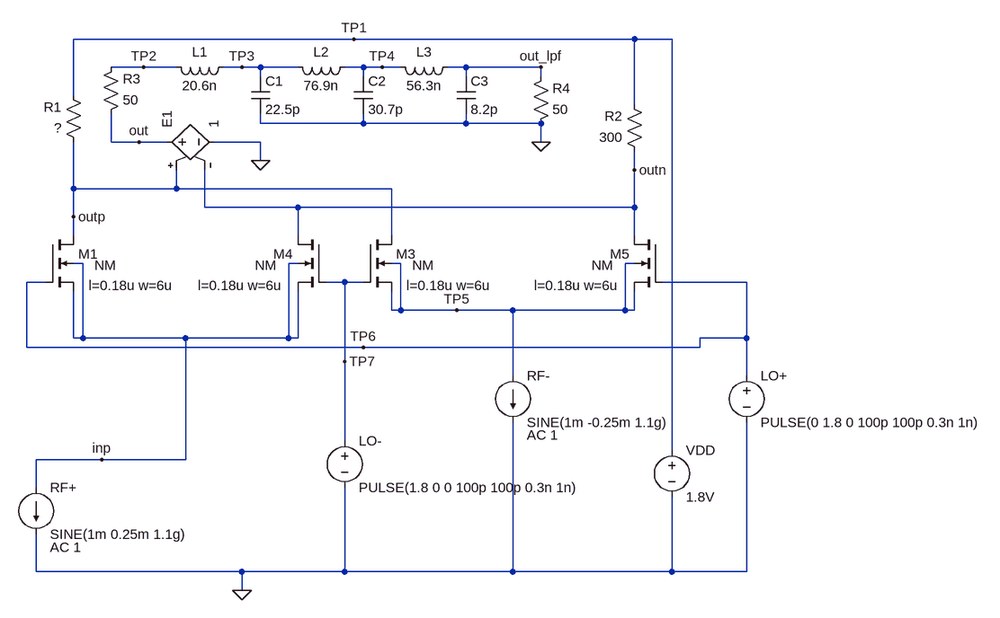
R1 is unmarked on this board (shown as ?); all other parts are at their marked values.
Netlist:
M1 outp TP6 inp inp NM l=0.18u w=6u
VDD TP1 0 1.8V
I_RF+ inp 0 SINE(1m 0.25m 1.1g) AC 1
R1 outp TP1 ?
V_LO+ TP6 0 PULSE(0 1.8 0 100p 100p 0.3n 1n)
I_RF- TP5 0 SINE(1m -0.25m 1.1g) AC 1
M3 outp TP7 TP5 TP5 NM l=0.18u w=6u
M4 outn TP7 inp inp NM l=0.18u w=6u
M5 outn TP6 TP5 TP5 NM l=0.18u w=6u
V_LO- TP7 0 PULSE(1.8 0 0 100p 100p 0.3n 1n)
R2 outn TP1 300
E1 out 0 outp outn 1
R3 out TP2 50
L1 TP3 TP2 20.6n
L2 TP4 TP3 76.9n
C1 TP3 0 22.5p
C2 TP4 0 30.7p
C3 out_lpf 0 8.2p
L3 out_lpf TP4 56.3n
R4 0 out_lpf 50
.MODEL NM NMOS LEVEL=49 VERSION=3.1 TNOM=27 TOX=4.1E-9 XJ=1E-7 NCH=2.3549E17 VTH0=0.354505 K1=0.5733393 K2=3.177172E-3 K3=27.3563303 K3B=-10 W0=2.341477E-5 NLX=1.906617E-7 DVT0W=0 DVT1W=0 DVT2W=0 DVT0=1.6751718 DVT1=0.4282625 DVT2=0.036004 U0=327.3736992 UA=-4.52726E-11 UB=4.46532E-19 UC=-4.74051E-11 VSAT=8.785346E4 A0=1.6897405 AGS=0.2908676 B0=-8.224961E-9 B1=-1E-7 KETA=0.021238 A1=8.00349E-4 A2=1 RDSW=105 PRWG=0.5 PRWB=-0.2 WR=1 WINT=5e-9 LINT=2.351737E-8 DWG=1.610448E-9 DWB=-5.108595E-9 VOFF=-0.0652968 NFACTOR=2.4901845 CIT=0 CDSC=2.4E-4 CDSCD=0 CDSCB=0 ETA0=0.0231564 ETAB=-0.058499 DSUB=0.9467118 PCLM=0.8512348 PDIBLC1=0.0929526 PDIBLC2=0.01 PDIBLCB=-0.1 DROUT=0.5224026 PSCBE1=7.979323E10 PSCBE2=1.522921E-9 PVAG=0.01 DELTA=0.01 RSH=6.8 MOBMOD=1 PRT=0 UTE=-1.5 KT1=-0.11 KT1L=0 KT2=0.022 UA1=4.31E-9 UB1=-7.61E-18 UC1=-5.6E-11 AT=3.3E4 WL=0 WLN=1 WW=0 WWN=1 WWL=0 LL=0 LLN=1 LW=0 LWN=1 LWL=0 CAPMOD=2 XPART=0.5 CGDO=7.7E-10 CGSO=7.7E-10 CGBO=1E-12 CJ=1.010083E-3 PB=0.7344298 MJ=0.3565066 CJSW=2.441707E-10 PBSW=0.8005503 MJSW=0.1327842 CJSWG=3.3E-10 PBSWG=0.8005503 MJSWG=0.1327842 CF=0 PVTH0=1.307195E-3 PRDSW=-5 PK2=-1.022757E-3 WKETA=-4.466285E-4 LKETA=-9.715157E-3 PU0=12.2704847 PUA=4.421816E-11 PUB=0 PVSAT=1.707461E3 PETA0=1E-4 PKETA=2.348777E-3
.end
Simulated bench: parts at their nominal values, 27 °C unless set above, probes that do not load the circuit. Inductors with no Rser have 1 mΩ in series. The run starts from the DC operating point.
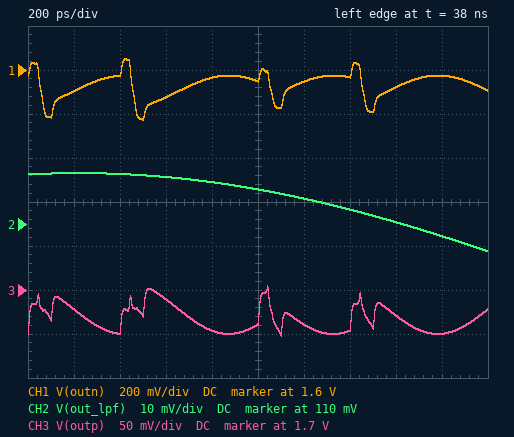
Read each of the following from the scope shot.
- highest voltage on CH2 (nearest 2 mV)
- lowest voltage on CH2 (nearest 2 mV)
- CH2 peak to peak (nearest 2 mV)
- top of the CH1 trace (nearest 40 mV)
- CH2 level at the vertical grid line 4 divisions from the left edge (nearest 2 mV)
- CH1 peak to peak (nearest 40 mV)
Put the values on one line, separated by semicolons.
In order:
122 mV; 104 mV; 18 mV; 1.64 V; 120 mV; 280 mV
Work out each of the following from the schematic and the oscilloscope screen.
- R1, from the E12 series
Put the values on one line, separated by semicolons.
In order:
120 Ω
